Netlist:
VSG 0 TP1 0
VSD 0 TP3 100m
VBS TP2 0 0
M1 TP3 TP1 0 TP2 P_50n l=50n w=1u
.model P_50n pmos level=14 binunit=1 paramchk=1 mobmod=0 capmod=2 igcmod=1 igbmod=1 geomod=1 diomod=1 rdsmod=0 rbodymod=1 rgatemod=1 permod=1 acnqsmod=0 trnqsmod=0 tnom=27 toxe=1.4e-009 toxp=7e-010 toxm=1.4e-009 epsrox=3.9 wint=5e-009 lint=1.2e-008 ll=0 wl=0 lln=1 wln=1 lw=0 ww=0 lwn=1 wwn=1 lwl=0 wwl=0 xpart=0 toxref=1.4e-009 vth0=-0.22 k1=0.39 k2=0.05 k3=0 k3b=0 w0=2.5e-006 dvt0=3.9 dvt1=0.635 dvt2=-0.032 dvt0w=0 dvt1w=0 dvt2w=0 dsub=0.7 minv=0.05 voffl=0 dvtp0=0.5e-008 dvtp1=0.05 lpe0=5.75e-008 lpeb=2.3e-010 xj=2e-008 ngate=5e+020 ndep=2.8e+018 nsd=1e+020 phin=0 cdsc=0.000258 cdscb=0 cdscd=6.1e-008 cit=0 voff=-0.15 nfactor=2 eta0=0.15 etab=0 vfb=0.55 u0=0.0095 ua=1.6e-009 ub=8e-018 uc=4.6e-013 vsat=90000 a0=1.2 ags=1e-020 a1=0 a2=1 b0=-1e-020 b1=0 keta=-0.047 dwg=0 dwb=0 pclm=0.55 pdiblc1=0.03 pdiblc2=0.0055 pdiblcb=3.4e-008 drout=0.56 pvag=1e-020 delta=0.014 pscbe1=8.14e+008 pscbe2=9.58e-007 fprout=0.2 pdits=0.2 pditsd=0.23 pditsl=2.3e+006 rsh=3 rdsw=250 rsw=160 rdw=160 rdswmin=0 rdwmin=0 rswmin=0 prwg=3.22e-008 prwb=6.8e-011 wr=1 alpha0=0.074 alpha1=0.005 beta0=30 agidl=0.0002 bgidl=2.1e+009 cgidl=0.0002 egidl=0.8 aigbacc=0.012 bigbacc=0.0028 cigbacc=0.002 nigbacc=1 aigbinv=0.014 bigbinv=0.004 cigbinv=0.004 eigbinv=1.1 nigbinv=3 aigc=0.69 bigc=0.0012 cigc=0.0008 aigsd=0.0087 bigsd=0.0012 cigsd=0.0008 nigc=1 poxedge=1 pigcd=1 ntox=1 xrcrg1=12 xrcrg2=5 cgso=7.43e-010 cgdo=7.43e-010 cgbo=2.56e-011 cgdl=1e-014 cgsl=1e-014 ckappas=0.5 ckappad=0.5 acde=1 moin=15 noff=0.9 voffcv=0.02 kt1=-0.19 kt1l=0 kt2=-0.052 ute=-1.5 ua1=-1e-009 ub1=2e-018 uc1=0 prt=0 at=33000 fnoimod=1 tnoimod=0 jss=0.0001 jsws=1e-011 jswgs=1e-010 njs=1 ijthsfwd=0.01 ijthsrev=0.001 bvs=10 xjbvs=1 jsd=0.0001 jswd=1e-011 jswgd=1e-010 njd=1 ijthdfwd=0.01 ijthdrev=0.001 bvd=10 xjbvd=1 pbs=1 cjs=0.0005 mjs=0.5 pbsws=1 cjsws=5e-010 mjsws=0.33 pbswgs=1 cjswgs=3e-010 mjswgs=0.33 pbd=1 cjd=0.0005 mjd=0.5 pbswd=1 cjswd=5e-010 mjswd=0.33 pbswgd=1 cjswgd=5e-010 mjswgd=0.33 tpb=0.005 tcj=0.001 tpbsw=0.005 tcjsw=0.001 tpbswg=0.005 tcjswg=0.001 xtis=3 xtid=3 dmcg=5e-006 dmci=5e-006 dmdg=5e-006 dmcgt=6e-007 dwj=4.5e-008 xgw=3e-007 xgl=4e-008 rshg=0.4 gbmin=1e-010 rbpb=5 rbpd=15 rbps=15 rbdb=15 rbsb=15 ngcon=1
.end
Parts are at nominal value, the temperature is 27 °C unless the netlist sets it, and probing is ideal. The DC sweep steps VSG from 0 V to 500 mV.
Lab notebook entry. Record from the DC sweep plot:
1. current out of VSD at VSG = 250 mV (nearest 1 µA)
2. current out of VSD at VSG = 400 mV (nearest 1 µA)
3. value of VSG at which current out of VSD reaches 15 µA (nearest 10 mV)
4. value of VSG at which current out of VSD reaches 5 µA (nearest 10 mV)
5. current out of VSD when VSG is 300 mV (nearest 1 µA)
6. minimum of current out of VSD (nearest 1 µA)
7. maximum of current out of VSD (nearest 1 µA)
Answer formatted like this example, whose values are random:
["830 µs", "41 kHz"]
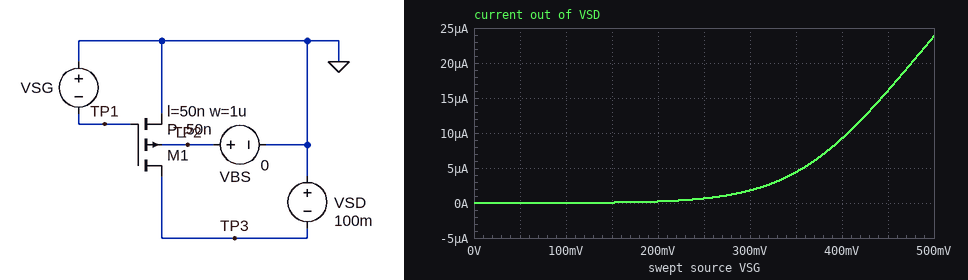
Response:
["1 µA", "9 µA", "440 mV", "360 mV", "2 µA", "0 A", "24 µA"]
